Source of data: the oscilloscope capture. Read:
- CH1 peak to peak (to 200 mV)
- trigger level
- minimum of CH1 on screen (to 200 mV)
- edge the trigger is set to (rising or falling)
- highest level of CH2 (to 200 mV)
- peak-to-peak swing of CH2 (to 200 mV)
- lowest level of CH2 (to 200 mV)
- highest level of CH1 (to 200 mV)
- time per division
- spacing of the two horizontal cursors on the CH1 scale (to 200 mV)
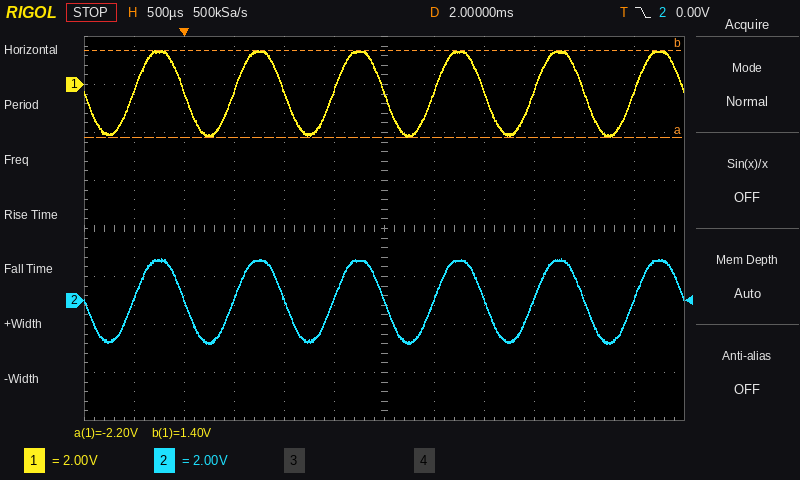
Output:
3.6 V
0.00 V
-2.2 V
falling
1.8 V
3.6 V
-1.8 V
1.4 V
500 µs
3.6 V
